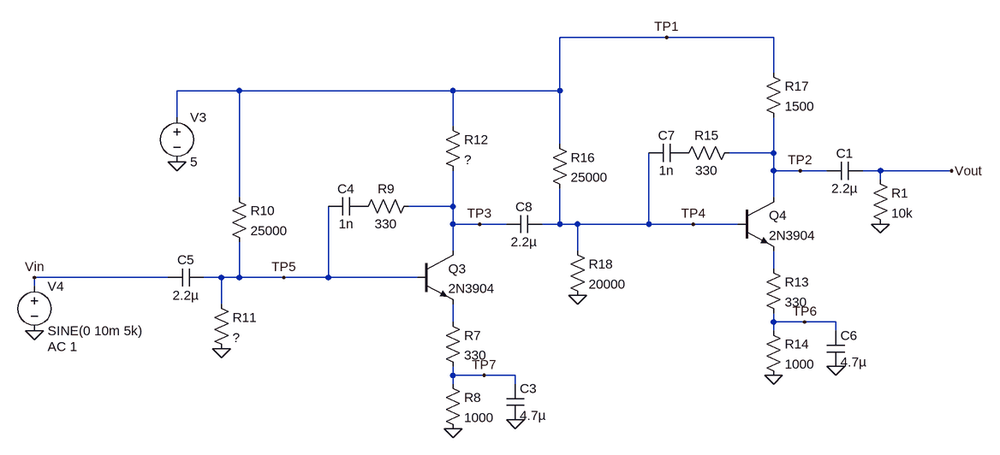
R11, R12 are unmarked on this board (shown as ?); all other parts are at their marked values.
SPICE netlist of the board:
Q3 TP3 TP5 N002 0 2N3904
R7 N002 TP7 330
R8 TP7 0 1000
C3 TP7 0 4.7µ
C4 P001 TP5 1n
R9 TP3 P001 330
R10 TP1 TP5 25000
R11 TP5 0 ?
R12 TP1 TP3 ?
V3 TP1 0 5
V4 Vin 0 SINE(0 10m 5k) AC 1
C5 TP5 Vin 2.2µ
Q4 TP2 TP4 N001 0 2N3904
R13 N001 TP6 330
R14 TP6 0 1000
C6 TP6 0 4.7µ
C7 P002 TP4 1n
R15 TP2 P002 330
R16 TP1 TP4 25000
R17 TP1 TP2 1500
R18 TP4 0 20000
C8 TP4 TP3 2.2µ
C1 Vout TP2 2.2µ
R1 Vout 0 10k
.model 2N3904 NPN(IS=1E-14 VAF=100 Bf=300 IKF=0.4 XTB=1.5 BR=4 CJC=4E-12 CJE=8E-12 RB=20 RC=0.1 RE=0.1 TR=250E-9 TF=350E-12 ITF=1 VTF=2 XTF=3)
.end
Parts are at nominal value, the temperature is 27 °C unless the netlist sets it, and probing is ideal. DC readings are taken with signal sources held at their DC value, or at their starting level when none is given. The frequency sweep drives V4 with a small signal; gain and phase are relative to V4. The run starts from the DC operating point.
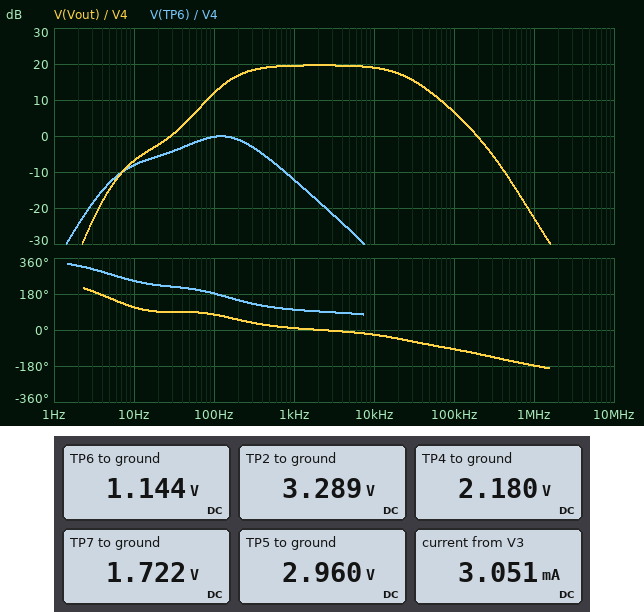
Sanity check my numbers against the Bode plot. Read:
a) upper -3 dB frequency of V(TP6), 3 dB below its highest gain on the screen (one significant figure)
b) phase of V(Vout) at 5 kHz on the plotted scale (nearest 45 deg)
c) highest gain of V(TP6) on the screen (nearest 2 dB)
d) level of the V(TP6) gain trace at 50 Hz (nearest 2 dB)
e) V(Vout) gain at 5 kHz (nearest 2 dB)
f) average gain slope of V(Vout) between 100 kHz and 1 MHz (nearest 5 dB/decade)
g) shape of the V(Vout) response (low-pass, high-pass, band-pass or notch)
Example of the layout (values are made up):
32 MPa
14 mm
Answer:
300 Hz
0 deg
0 dB
-2 dB
20 dB
-30 dB/decade
band-pass
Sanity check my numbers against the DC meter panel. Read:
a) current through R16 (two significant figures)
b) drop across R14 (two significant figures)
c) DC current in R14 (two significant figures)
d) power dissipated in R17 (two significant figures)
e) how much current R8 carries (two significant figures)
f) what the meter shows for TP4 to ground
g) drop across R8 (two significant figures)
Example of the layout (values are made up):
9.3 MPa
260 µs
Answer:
110 µA
1.1 V
1.1 mA
2.0 mW
1.7 mA
2.180 V
1.7 V
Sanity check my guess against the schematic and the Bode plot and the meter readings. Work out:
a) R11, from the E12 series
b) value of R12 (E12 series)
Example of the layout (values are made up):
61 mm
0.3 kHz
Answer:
39 kΩ
1 kΩ
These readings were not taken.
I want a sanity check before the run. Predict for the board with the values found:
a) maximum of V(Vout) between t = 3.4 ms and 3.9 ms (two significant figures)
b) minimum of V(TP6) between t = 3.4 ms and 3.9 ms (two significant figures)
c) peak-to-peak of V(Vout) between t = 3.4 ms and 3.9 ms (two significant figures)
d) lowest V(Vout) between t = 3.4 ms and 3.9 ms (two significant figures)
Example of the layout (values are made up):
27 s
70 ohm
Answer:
94 mV
1.1 V
190 mV
-94 mV
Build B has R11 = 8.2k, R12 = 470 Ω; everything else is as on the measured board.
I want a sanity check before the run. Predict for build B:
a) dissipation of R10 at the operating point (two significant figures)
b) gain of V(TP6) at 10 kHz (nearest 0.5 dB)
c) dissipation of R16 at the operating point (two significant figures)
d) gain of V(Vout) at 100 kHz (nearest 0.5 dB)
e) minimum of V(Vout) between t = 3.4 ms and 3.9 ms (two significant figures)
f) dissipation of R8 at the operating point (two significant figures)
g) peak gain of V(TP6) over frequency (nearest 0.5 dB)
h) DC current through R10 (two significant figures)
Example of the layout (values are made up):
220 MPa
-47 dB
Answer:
570 µW
-39.5 dB
320 µW
3.5 dB
-42 mV
200 µW
-7.0 dB
150 µA
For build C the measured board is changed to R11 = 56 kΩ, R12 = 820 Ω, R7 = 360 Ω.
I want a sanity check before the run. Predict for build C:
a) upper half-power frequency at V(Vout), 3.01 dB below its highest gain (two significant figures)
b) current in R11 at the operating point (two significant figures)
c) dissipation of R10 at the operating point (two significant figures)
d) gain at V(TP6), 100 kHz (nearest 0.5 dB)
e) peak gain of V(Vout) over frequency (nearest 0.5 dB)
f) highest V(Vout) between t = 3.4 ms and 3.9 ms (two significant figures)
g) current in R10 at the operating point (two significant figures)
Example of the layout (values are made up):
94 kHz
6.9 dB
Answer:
28 kHz
60 µA
110 µW
-63.0 dB
17.5 dB
73 mV
66 µA
